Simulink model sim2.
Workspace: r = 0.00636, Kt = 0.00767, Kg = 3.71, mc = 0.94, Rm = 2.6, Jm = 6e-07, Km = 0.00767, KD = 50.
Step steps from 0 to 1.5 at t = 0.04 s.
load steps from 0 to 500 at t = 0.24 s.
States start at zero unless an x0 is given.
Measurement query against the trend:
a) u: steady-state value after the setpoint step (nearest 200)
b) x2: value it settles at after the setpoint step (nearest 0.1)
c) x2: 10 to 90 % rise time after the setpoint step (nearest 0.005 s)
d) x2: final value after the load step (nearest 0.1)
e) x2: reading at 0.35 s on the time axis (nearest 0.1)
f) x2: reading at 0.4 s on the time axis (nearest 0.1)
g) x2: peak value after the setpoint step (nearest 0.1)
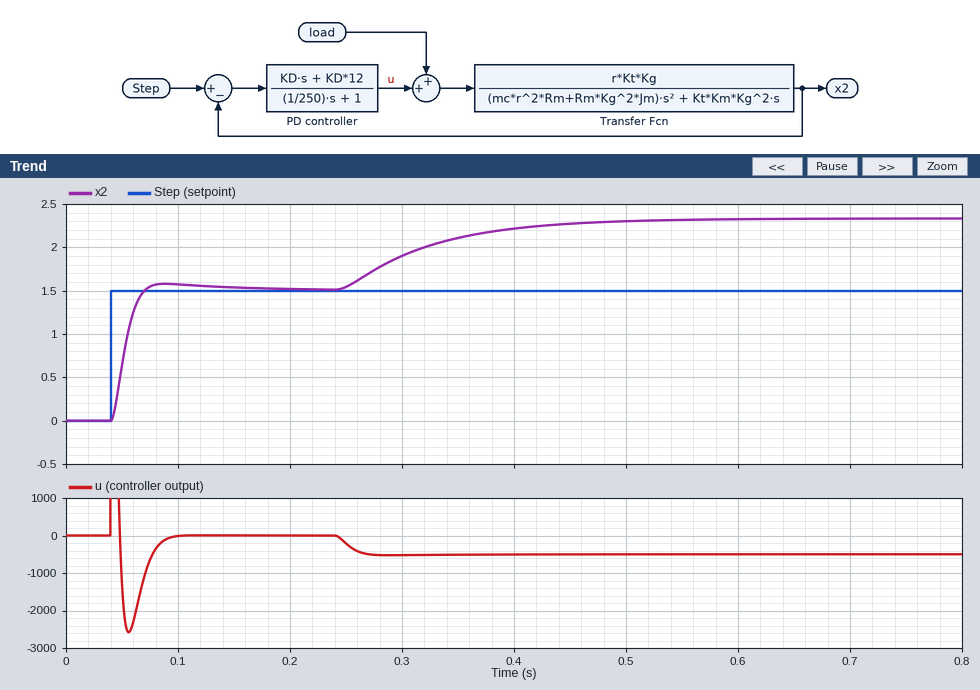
0
1.5
0.020 s
2.3
2.1
2.2
1.6
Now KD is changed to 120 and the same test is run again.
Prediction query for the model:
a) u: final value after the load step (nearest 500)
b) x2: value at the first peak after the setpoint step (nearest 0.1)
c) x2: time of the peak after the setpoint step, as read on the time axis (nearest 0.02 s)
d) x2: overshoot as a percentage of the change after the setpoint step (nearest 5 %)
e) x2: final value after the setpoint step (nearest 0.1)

-500
1.7
0.06 s
15 %
1.5
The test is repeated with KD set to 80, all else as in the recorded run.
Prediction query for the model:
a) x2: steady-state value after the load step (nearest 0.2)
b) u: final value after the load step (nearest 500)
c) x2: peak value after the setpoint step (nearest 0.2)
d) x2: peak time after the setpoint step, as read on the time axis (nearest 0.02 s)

2.0
-500
1.6
0.06 s
